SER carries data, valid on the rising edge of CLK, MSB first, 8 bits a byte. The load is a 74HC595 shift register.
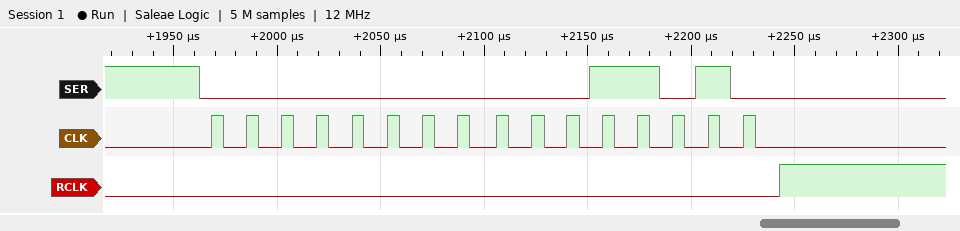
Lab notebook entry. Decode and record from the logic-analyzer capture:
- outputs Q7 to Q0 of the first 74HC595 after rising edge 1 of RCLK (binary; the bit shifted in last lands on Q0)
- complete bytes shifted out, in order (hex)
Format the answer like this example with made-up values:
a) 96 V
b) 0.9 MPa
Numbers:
a) 00011010
b) 0x00 0x1A
